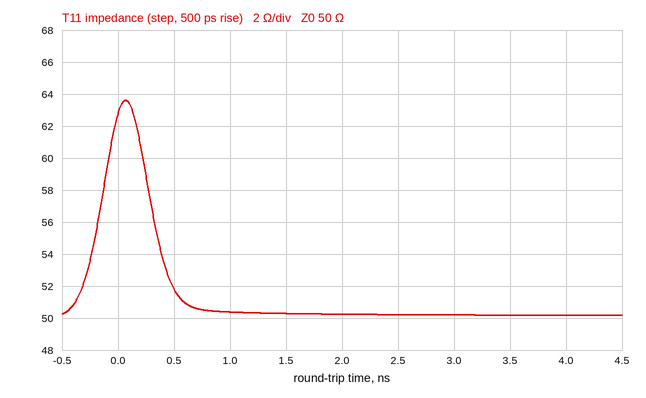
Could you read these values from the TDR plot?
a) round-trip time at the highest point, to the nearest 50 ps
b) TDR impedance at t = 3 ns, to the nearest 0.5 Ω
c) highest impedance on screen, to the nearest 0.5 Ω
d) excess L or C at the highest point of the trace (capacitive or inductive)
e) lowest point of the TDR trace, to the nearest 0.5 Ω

50 ps
50.0 Ω
63.5 Ω
inductive
50.0 Ω
